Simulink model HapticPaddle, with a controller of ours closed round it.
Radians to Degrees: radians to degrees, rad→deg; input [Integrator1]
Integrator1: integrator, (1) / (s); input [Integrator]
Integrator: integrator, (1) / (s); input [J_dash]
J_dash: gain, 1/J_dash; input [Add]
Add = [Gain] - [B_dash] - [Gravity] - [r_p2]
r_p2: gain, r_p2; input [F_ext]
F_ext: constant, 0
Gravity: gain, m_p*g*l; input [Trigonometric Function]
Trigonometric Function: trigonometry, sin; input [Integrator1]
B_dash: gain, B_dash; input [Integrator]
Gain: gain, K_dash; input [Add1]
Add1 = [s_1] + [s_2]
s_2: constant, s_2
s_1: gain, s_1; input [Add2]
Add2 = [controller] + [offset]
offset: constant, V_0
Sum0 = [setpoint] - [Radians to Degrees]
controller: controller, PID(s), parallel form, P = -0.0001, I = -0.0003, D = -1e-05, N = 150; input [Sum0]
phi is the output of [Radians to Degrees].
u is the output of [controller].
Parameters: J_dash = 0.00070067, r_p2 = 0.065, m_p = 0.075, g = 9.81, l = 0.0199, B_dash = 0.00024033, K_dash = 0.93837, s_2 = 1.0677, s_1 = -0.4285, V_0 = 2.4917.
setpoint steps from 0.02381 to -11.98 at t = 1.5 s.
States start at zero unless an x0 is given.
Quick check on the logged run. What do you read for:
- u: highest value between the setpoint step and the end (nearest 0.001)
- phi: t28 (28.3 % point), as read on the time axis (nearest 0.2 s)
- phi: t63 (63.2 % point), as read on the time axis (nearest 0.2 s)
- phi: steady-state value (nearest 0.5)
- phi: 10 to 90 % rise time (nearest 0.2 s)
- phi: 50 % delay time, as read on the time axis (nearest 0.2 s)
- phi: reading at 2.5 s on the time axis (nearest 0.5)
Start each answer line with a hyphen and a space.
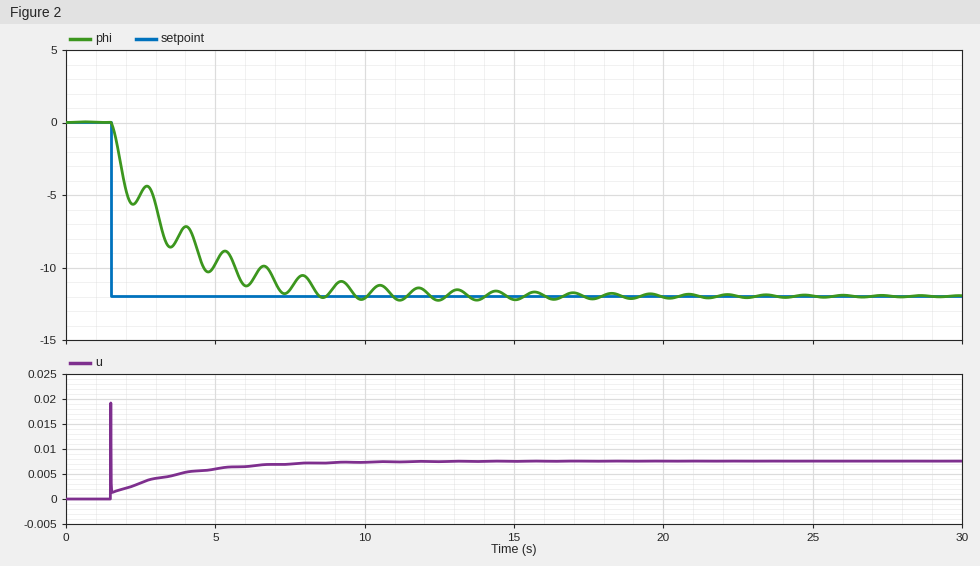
- 0.019
- 1.8 s
- 3.2 s
- -12.0
- 4.2 s
- 3.0 s
- -5.0
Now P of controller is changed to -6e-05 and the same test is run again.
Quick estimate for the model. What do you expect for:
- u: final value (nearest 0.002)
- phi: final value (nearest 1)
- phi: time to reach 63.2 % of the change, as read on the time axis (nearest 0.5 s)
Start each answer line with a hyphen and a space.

- 0.008
- -12
- 3.5 s
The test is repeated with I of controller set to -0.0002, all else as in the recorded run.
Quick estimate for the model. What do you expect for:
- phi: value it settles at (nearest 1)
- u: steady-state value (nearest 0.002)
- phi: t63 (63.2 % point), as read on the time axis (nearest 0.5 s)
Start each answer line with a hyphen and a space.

- -12
- 0.008
- 4.5 s
